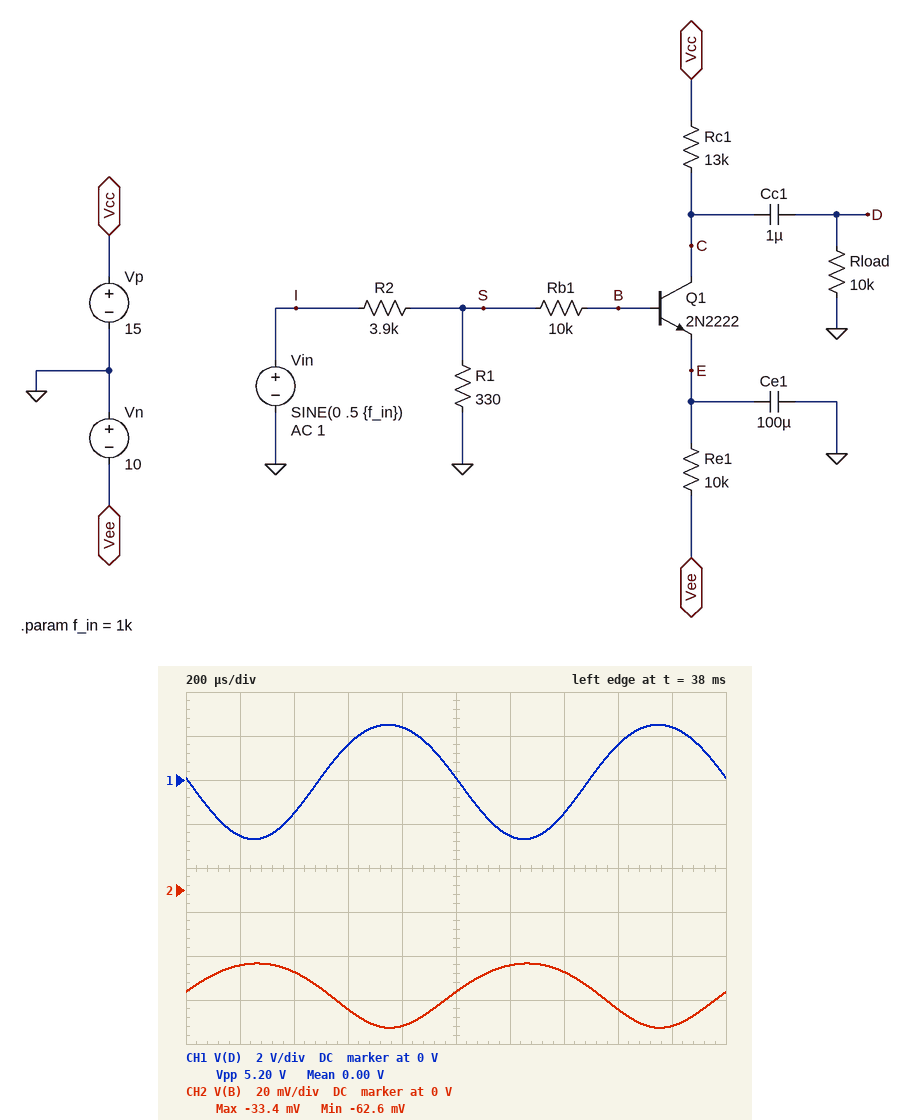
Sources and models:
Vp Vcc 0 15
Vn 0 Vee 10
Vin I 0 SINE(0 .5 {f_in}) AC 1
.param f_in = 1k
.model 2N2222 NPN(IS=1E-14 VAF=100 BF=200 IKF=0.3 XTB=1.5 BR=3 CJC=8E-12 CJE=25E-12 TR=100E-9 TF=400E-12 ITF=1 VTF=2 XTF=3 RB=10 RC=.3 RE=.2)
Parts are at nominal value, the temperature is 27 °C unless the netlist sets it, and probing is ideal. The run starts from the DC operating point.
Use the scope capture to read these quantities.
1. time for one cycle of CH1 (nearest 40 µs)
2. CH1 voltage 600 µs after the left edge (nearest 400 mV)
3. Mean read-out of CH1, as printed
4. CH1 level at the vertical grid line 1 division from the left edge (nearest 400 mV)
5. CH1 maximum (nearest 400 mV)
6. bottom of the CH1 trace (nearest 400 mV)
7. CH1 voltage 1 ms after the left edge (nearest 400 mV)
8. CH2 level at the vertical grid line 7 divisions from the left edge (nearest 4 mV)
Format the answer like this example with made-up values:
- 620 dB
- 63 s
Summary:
- 1.00 ms
- 1.6 V
- 0.00 V
- -2.4 V
- 2.4 V
- -2.8 V
- 0 V
- -36 mV
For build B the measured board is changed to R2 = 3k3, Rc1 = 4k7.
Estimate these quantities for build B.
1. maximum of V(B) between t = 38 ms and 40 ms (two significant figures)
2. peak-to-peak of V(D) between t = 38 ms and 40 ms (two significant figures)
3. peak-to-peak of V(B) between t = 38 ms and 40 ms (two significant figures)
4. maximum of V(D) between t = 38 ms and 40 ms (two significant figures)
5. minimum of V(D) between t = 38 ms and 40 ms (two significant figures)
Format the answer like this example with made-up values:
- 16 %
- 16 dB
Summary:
- -27 mV
- 3.6 V
- 36 mV
- 1.7 V
- -1.9 V
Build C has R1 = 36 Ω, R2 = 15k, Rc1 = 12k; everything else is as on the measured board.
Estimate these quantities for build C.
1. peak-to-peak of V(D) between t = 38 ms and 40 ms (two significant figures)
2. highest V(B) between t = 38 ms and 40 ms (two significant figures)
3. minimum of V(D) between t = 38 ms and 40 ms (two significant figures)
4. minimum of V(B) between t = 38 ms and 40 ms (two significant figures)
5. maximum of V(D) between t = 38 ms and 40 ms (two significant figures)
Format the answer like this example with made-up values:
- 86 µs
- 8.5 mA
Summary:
- 160 mV
- -44 mV
- -81 mV
- -45 mV
- 81 mV
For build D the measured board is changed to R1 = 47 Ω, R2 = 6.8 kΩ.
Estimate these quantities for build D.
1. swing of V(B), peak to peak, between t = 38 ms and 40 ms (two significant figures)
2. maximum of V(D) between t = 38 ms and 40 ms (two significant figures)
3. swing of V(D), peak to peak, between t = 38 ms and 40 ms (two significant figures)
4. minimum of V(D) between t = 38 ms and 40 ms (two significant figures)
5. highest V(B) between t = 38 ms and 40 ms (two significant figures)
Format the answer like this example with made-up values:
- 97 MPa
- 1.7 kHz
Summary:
- 2.5 mV
- 240 mV
- 480 mV
- -240 mV
- -44 mV
